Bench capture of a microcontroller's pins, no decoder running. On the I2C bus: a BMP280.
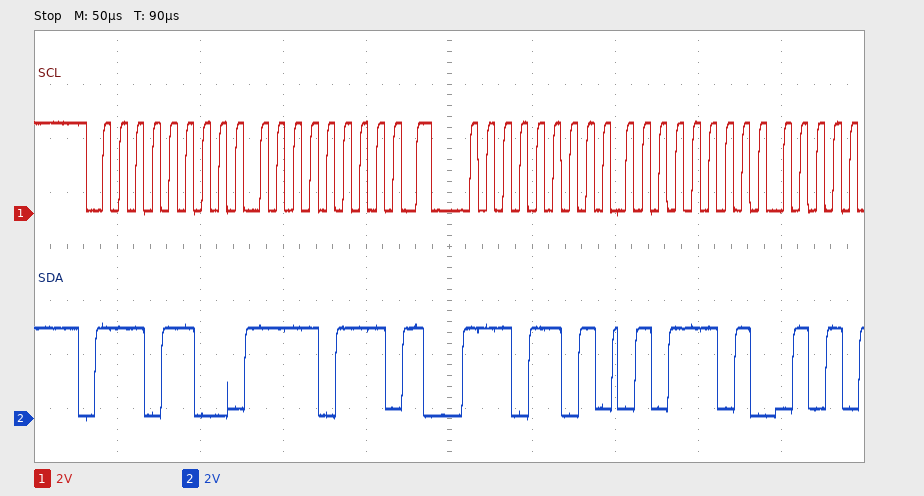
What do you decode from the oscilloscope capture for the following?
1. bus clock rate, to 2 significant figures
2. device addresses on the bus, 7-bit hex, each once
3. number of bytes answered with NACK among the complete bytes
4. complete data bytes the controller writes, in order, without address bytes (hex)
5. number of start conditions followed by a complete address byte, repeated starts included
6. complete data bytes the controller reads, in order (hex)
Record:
100 kHz
0x76
0
F7
2
5D
